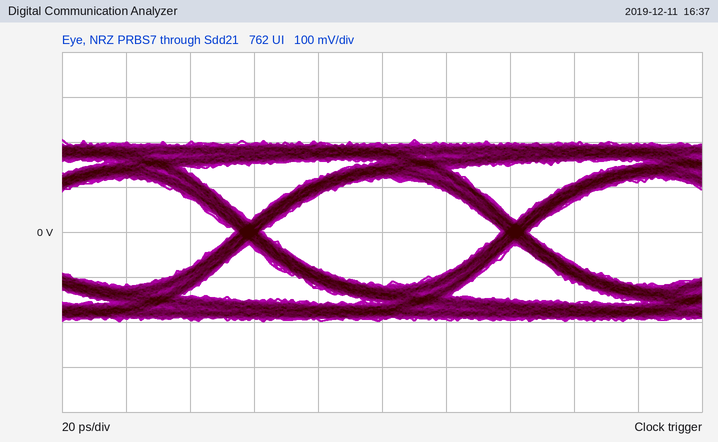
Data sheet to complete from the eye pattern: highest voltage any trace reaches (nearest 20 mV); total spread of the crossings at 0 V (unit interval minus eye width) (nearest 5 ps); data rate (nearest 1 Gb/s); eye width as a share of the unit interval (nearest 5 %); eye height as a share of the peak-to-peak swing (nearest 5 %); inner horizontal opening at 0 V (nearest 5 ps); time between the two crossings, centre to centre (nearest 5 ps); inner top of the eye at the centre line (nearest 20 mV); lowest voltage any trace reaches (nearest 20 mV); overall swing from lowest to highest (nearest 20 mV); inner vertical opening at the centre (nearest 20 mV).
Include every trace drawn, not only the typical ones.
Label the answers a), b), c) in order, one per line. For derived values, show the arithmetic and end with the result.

a) 200 mV
b) 10 ps
c) 12 Gb/s
d) 75 ps / 85 ps ≈ 88.2 %, so 90 % to the nearest 5 %
e) 240 mV / 400 mV ≈ 60 %
f) 75 ps
g) 85 ps
h) 120 mV
i) -200 mV
j) 400 mV
k) 240 mV
